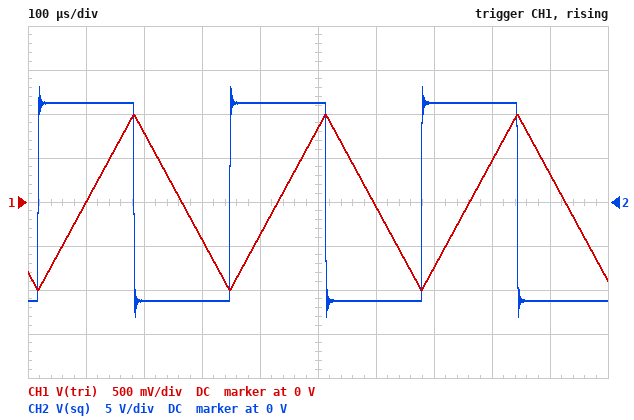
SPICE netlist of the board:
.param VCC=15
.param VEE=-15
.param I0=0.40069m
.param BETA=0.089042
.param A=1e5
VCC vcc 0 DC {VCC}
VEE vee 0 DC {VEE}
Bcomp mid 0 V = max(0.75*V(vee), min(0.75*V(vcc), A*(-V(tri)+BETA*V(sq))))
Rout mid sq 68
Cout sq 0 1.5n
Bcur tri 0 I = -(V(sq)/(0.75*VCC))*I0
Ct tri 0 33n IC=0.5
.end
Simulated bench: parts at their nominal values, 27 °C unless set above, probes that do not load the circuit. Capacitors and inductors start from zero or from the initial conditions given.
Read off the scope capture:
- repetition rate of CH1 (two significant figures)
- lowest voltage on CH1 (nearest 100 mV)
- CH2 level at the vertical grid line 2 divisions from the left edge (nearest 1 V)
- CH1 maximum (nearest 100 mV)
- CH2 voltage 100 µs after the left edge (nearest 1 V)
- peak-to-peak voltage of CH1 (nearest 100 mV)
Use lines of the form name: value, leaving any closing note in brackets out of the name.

repetition rate of CH1: 3.0 kHz
lowest voltage on CH1: -1.0 V
CH2 level at the vertical grid line 2 divisions from the left edge: -11 V
CH1 maximum: 1.0 V
CH2 voltage 100 µs after the left edge: 11 V
peak-to-peak voltage of CH1: 2.0 V
